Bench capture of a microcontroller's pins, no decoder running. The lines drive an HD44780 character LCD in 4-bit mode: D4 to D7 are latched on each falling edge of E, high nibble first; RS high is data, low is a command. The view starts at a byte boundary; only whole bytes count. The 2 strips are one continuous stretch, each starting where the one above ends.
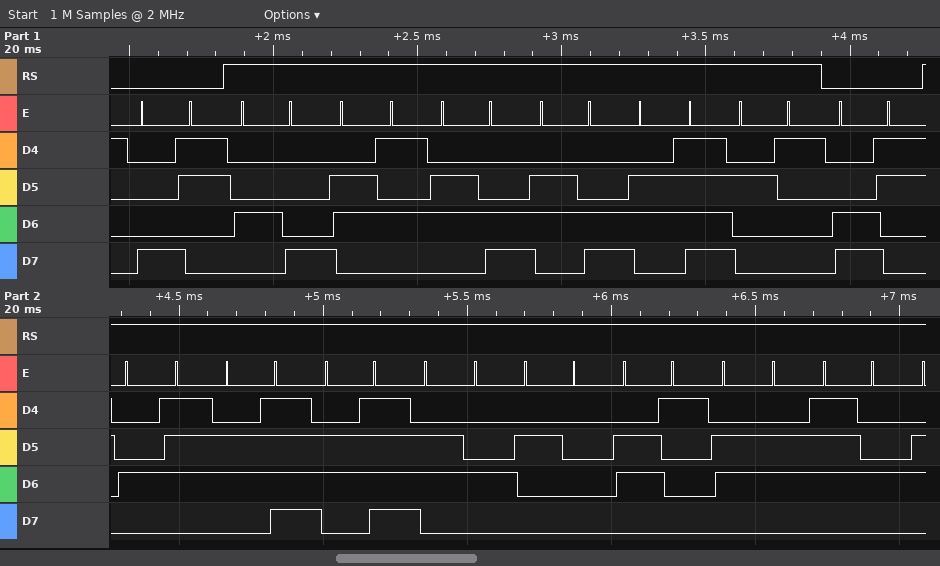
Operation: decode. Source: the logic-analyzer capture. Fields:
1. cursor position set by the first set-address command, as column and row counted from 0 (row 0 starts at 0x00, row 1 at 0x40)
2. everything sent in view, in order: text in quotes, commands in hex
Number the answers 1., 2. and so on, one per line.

1. column 3, row 0
2. 0x83 "Hello!" 0xC3 "Good aft"
